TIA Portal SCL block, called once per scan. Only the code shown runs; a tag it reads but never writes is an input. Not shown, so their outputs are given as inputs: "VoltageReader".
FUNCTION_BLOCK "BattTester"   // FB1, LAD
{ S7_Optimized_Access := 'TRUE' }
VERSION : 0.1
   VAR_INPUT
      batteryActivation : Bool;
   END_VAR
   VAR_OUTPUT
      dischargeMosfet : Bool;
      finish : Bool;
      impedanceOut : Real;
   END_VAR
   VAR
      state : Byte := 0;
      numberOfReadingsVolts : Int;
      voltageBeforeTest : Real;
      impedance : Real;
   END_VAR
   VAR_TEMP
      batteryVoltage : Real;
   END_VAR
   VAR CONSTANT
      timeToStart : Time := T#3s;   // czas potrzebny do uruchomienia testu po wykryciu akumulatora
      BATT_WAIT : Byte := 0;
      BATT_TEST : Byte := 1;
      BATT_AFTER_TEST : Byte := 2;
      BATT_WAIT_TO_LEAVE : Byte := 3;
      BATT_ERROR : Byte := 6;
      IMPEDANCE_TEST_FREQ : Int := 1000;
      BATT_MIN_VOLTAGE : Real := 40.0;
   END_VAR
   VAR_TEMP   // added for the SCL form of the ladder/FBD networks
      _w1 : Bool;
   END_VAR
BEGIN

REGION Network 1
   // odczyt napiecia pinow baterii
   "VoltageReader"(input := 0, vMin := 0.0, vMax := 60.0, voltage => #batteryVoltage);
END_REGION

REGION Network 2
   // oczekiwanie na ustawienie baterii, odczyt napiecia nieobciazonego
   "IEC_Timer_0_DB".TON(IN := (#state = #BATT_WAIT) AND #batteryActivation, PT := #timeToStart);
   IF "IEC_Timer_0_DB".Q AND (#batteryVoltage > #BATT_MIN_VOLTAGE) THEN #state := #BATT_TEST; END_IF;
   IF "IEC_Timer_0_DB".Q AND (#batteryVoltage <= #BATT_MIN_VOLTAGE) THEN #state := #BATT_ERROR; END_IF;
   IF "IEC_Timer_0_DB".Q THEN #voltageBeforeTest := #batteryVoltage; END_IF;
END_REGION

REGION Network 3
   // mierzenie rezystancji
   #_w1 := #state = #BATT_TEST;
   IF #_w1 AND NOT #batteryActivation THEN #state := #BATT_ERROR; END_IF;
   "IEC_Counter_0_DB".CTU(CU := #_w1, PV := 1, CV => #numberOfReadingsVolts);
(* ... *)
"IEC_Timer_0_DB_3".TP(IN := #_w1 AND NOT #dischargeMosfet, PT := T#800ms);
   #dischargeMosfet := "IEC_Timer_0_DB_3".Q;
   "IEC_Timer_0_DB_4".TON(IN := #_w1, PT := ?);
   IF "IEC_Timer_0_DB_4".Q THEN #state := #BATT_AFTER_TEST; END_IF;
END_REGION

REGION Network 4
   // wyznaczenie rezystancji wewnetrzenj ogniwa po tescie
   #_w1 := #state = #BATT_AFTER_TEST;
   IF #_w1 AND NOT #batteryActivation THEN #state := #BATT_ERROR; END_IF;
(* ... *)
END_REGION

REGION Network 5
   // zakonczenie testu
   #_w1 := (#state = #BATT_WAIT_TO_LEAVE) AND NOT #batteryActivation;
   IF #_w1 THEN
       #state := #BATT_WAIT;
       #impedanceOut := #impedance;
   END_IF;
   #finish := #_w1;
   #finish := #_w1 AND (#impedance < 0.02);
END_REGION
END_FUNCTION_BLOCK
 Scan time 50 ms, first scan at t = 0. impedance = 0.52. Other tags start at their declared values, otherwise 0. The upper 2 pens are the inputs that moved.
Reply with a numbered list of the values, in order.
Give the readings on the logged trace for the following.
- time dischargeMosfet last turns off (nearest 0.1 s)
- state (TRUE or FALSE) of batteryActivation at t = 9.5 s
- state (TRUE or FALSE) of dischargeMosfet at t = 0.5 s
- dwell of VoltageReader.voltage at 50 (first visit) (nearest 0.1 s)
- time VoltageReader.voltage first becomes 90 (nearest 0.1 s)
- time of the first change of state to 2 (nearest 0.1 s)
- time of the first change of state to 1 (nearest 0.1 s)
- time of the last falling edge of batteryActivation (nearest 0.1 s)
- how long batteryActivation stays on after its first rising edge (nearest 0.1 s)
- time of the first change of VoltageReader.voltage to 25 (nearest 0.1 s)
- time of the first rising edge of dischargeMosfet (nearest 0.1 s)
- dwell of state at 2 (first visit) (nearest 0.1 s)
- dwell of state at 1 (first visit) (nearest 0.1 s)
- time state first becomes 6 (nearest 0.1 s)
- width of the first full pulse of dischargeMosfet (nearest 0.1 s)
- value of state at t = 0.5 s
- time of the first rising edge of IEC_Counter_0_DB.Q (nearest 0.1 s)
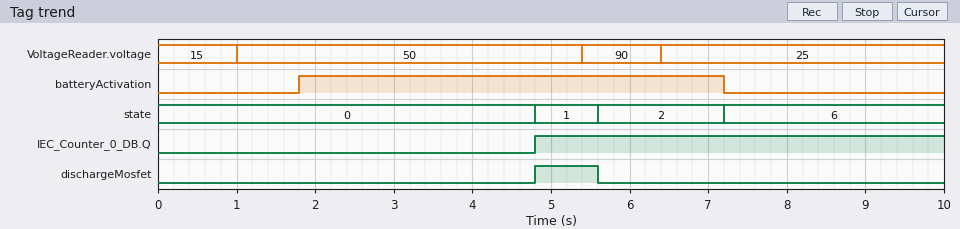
1. 5.6 s
2. FALSE
3. FALSE
4. 4.4 s
5. 5.4 s
6. 5.6 s
7. 4.8 s
8. 7.2 s
9. 5.4 s
10. 6.4 s
11. 4.8 s
12. 1.6 s
13. 0.8 s
14. 7.2 s
15. 0.8 s
16. 0
17. 4.8 s
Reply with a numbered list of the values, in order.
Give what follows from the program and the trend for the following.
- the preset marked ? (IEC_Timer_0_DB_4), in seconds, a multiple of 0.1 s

1. 0.8 s
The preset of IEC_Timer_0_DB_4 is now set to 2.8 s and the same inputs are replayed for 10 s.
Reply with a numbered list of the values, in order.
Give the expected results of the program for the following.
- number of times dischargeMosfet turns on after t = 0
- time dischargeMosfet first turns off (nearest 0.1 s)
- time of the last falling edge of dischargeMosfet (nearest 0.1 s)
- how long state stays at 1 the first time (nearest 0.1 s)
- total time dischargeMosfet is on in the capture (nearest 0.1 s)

1. 3
2. 5.6 s
3. 7.3 s
4. 2.4 s
5. 2.4 s
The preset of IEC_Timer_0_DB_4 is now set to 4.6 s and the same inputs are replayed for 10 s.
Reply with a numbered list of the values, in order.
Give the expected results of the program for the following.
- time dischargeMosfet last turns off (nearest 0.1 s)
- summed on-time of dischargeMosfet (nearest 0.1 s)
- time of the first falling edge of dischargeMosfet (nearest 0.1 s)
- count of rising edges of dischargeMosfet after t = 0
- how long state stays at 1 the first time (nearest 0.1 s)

1. 7.3 s
2. 2.4 s
3. 5.6 s
4. 3
5. 2.4 s
